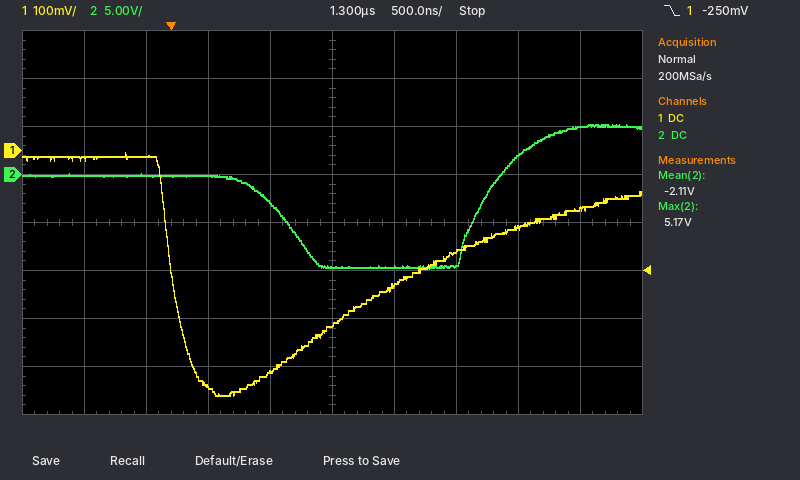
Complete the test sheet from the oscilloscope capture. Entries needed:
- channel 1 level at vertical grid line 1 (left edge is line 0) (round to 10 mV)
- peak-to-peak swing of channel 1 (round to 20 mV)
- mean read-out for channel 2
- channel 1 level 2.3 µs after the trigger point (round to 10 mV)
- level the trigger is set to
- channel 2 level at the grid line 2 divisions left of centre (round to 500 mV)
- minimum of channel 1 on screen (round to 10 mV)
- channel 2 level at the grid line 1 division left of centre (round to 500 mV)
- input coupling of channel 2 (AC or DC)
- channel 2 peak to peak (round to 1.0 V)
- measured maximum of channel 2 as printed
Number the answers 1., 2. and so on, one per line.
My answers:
1. -20 mV
2. 500 mV
3. -2.11 V
4. -210 mV
5. -250 mV
6. 0.0 V
7. -510 mV
8. -3.0 V
9. DC
10. 15.0 V
11. 5.17 V
